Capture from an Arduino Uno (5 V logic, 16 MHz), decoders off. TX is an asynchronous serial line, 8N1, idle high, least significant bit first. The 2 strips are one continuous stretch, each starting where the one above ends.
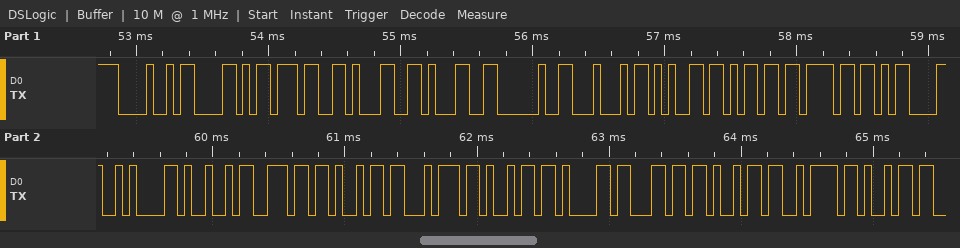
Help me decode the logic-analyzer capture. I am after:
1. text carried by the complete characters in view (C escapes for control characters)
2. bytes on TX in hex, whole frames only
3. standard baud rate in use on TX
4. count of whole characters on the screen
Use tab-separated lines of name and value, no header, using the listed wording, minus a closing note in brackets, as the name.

text carried by the complete characters in view	"HX711 Demo\r\nInitializi"
bytes on TX in hex, whole frames only	48 58 37 31 31 20 44 65 6D 6F 0D 0A 49 6E 69 74 69 61 6C 69 7A 69
standard baud rate in use on TX	19200 baud
count of whole characters on the screen	22
